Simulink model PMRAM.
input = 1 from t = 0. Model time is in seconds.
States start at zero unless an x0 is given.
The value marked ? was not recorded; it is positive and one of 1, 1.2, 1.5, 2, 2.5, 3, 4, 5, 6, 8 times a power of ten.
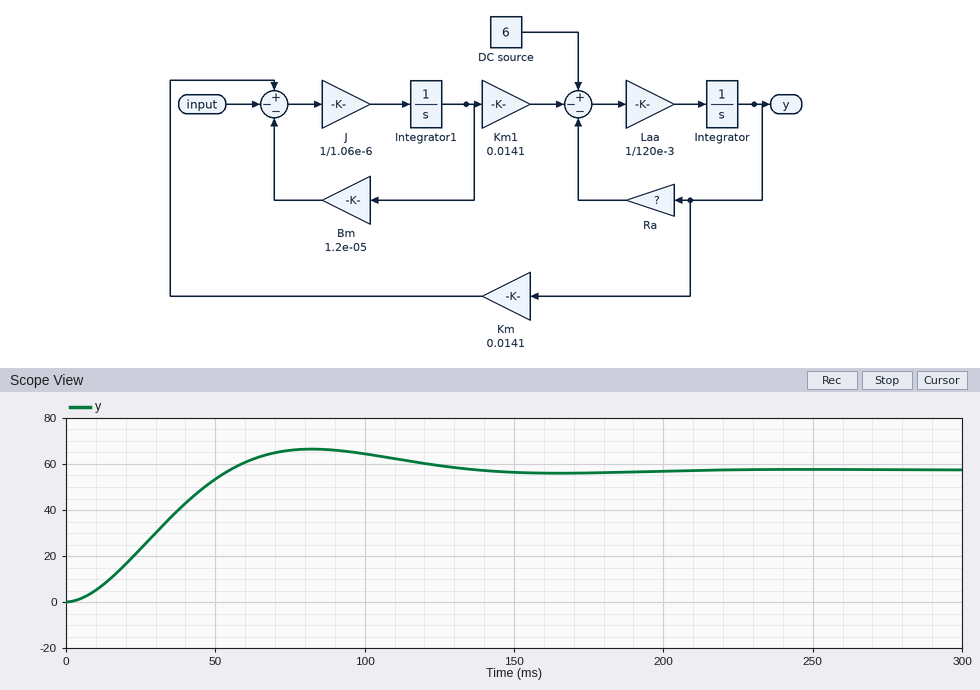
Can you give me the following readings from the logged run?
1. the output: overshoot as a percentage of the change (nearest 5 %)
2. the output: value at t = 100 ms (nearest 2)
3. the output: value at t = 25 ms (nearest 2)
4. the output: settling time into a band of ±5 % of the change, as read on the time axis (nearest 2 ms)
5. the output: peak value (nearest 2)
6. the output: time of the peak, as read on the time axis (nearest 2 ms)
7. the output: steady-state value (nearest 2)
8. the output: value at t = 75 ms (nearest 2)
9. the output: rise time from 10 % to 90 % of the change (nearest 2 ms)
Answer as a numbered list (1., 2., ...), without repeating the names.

1. 15 %
2. 64
3. 24
4. 120 ms
5. 66
6. 82 ms
7. 58
8. 66
9. 38 ms
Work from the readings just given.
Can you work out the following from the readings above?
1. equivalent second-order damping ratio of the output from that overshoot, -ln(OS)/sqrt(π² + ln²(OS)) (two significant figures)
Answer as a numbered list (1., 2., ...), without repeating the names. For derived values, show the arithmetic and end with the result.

1. ln(0.15) = -1.897; 1.897 / sqrt(9.870 + 3.599) = 0.52
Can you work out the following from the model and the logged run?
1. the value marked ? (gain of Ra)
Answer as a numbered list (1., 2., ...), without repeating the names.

1. 4
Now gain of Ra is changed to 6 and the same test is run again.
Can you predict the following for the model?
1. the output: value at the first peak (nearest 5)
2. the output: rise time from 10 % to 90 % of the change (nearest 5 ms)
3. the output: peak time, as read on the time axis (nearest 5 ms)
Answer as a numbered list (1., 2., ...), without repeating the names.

1. 55
2. 45 ms
3. 90 ms
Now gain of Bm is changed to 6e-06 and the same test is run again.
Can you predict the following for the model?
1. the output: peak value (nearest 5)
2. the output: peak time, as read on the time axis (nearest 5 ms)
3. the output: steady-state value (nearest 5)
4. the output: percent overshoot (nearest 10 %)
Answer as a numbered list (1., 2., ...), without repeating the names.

1. 75
2. 85 ms
3. 65
4. 20 %
